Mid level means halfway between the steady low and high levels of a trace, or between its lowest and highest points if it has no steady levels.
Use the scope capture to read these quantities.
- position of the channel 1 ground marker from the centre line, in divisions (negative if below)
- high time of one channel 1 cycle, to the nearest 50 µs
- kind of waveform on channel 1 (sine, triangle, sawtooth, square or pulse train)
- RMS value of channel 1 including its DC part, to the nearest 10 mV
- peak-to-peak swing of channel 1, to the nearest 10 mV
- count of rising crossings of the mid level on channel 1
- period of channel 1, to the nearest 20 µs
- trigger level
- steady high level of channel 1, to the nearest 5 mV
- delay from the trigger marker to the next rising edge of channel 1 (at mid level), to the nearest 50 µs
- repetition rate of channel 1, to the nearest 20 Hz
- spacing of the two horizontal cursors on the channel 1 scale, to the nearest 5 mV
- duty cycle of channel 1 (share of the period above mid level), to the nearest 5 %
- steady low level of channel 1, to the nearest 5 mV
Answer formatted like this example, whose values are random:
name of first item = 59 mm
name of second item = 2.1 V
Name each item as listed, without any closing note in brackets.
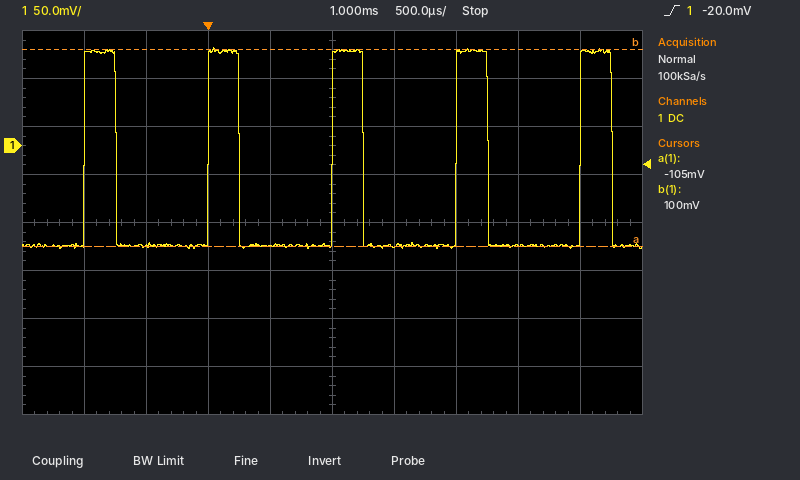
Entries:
position of the channel 1 ground marker from the centre line, in divisions = +1.6 div
high time of one channel 1 cycle, to the nearest 50 µs = 250 µs
kind of waveform on channel 1 = pulse train
RMS value of channel 1 including its DC part, to the nearest 10 mV = 100 mV
peak-to-peak swing of channel 1, to the nearest 10 mV = 210 mV
count of rising crossings of the mid level on channel 1 = 5
period of channel 1, to the nearest 20 µs = 1.00 ms
trigger level = -20.0 mV
steady high level of channel 1, to the nearest 5 mV = 100 mV
delay from the trigger marker to the next rising edge of channel 1 (at mid level), to the nearest 50 µs = 1.00 ms
repetition rate of channel 1, to the nearest 20 Hz = 1.00 kHz
spacing of the two horizontal cursors on the channel 1 scale, to the nearest 5 mV = 205 mV
duty cycle of channel 1 (share of the period above mid level), to the nearest 5 % = 25 %
steady low level of channel 1, to the nearest 5 mV = -105 mV
